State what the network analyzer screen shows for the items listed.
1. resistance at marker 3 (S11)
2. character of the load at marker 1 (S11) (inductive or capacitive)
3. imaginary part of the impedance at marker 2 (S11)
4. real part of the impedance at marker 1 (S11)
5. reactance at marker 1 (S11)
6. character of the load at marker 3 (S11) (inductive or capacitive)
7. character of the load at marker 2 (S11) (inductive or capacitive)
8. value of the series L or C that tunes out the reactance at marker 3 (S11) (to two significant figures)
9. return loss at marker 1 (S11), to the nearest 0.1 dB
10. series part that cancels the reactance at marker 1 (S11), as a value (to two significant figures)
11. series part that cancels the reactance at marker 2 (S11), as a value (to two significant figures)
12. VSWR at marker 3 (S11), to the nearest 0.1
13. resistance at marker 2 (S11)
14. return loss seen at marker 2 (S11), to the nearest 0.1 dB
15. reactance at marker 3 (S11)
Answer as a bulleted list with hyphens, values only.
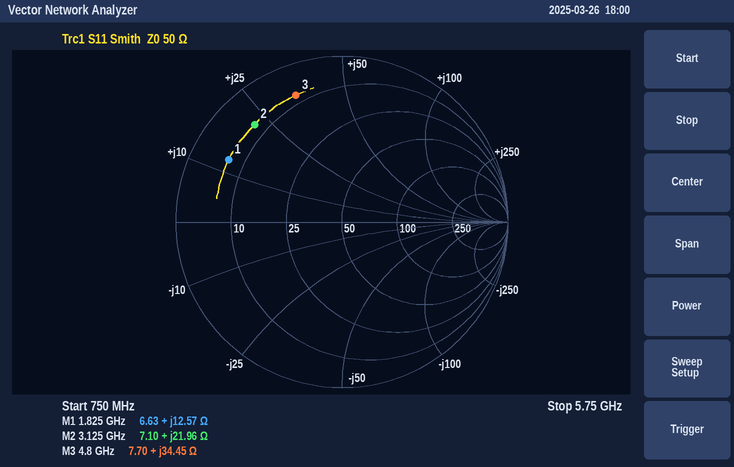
- 7.70 Ω
- inductive
- +21.96 Ω
- 6.63 Ω
- +12.57 Ω
- inductive
- inductive
- 960 fF
- 2.2 dB
- 6.9 pF
- 2.3 pF
- 9.6
- 7.10 Ω
- 2.1 dB
- +34.45 Ω
